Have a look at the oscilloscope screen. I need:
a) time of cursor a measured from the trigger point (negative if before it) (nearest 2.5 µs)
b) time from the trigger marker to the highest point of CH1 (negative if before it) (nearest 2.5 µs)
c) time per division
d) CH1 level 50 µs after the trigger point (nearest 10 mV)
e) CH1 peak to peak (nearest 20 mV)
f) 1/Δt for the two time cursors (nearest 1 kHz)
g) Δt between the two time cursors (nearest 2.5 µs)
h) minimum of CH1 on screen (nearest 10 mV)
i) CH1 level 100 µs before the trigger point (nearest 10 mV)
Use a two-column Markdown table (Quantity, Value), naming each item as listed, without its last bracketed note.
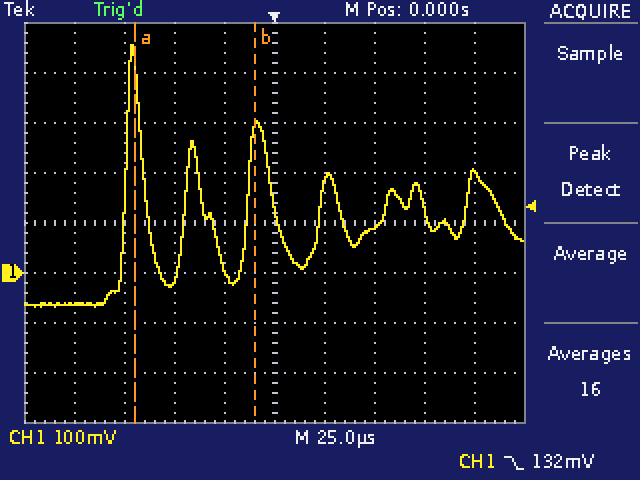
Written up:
| Quantity | Value |
|---|---|
| time of cursor a measured from the trigger point (negative if before it) | -70.0 µs |
| time from the trigger marker to the highest point of CH1 (negative if before it) | -70.0 µs |
| time per division | 25 µs |
| CH1 level 50 µs after the trigger point | 90 mV |
| CH1 peak to peak | 520 mV |
| 1/Δt for the two time cursors | 17 kHz |
| Δt between the two time cursors | 60.0 µs |
| minimum of CH1 on screen | -70 mV |
| CH1 level 100 µs before the trigger point | -60 mV |
